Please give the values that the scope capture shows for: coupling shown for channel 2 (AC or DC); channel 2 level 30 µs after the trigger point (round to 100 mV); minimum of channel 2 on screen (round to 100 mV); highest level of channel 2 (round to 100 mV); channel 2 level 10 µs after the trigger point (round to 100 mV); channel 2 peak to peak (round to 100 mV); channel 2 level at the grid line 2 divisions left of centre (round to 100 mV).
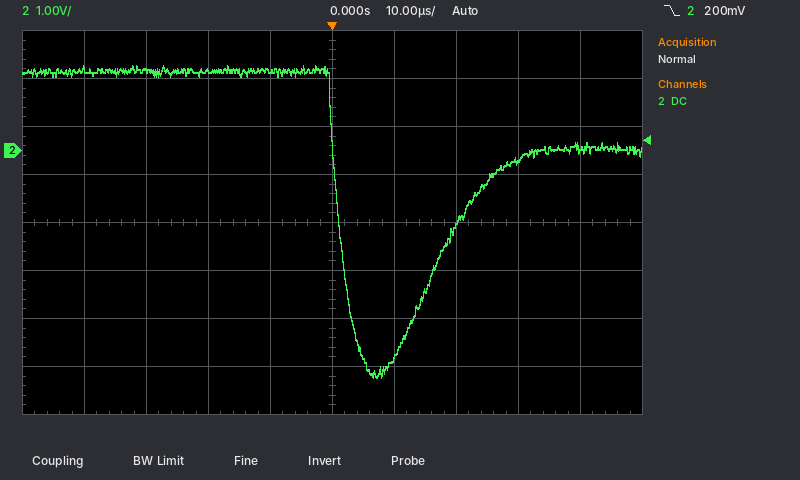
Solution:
DC
-200 mV
-4.7 V
1.8 V
-4.3 V
6.5 V
1.7 V
